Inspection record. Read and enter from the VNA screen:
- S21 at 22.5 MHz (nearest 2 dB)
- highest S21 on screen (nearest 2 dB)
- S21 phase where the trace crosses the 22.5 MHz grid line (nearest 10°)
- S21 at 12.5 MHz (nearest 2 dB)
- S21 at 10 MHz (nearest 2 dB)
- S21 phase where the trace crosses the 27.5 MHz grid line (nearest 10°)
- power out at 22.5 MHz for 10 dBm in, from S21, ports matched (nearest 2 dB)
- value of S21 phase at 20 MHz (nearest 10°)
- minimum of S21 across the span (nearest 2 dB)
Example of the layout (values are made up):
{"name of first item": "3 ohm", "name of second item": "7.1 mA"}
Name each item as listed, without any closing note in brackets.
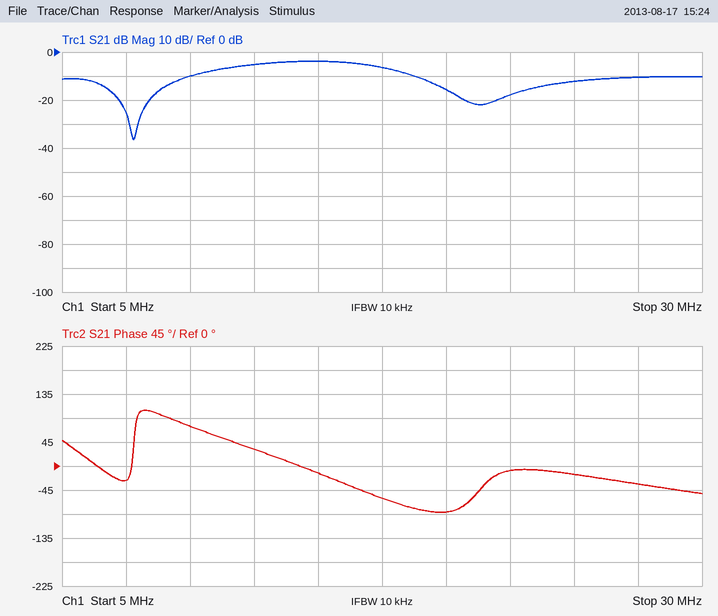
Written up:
{"S21 at 22.5 MHz": "-18 dB", "highest S21 on screen": "-4 dB", "S21 phase where the trace crosses the 22.5 MHz grid line": "-10°", "S21 at 12.5 MHz": "-6 dB", "S21 at 10 MHz": "-10 dB", "S21 phase where the trace crosses the 27.5 MHz grid line": "-30°", "power out at 22.5 MHz for 10 dBm in, from S21, ports matched": "-8 dBm", "value of S21 phase at 20 MHz": "-90°", "minimum of S21 across the span": "-36 dB"}
